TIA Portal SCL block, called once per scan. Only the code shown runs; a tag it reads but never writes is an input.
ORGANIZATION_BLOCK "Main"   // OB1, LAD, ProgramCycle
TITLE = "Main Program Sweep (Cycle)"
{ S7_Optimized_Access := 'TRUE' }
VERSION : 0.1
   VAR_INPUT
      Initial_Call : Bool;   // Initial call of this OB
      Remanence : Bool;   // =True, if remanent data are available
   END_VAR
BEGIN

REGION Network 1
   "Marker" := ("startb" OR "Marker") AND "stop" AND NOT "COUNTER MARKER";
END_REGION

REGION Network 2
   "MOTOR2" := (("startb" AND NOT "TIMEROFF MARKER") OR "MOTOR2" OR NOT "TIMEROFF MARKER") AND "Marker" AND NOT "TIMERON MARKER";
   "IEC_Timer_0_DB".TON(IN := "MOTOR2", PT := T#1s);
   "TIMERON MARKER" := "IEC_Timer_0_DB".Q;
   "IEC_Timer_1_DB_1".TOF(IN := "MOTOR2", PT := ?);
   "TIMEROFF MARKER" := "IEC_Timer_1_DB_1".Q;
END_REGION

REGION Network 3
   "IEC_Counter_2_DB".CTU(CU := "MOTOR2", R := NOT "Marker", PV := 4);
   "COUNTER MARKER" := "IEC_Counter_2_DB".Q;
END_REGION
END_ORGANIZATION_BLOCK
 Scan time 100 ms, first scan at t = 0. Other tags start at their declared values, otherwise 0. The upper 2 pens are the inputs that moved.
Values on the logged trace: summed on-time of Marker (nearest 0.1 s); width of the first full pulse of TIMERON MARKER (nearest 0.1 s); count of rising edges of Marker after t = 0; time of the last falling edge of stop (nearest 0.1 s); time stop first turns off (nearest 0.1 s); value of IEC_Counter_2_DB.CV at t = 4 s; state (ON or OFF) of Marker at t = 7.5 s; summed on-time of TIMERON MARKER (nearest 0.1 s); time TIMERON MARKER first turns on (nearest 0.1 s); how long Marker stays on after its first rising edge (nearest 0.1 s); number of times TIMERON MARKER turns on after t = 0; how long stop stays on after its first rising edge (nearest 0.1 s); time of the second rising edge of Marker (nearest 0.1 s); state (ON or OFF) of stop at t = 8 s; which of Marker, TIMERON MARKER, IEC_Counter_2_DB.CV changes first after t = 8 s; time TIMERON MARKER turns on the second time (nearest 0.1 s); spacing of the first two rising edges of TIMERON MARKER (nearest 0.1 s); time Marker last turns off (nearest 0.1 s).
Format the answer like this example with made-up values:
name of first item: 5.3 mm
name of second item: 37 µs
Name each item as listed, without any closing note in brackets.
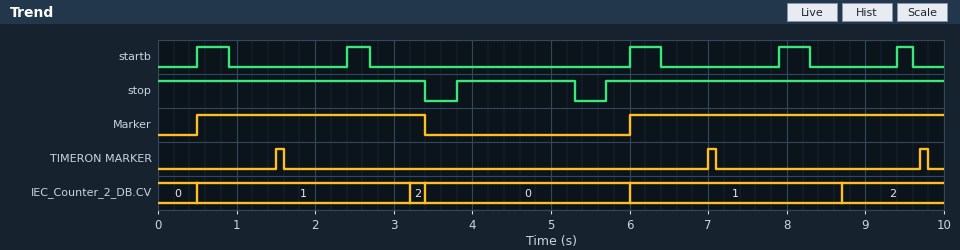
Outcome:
summed on-time of Marker: 6.9 s
width of the first full pulse of TIMERON MARKER: 0.1 s
count of rising edges of Marker after t = 0: 2
time of the last falling edge of stop: 5.3 s
time stop first turns off: 3.4 s
value of IEC_Counter_2_DB.CV at t = 4 s: 0
state (ON or OFF) of Marker at t = 7.5 s: ON
summed on-time of TIMERON MARKER: 0.3 s
time TIMERON MARKER first turns on: 1.5 s
how long Marker stays on after its first rising edge: 2.9 s
number of times TIMERON MARKER turns on after t = 0: 3
how long stop stays on after its first rising edge: 1.5 s
time of the second rising edge of Marker: 6.0 s
state (ON or OFF) of stop at t = 8 s: ON
which of Marker, TIMERON MARKER, IEC_Counter_2_DB.CV changes first after t = 8 s: IEC_Counter_2_DB.CV
time TIMERON MARKER turns on the second time: 7.0 s
spacing of the first two rising edges of TIMERON MARKER: 5.5 s
time Marker last turns off: 3.4 s
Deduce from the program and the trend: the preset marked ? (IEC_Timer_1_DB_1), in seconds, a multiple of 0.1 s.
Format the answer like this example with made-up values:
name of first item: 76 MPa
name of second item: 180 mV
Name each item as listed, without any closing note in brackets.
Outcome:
the preset marked ? (IEC_Timer_1_DB_1), in seconds, a multiple of 0.1 s: 1.5 s
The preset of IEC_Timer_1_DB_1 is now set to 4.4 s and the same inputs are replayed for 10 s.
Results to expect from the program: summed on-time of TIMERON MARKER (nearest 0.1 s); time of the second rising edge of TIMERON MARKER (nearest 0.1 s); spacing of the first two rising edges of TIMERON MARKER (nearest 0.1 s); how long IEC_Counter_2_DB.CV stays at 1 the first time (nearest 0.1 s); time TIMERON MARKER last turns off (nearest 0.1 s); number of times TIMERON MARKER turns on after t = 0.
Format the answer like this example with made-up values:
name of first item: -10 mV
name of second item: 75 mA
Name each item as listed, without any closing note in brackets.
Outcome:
summed on-time of TIMERON MARKER: 0.2 s
time of the second rising edge of TIMERON MARKER: 7.1 s
spacing of the first two rising edges of TIMERON MARKER: 5.6 s
how long IEC_Counter_2_DB.CV stays at 1 the first time: 2.9 s
time TIMERON MARKER last turns off: 7.2 s
number of times TIMERON MARKER turns on after t = 0: 2
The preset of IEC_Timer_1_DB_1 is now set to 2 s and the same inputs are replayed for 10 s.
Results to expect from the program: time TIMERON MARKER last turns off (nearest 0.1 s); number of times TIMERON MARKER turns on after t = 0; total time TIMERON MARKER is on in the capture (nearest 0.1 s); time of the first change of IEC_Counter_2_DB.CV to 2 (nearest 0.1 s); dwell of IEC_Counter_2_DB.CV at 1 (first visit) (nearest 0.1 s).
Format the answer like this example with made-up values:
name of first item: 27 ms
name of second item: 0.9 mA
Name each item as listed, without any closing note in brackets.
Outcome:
time TIMERON MARKER last turns off: 7.1 s
number of times TIMERON MARKER turns on after t = 0: 2
total time TIMERON MARKER is on in the capture: 0.2 s
time of the first change of IEC_Counter_2_DB.CV to 2: 9.2 s
dwell of IEC_Counter_2_DB.CV at 1 (first visit): 2.9 s
